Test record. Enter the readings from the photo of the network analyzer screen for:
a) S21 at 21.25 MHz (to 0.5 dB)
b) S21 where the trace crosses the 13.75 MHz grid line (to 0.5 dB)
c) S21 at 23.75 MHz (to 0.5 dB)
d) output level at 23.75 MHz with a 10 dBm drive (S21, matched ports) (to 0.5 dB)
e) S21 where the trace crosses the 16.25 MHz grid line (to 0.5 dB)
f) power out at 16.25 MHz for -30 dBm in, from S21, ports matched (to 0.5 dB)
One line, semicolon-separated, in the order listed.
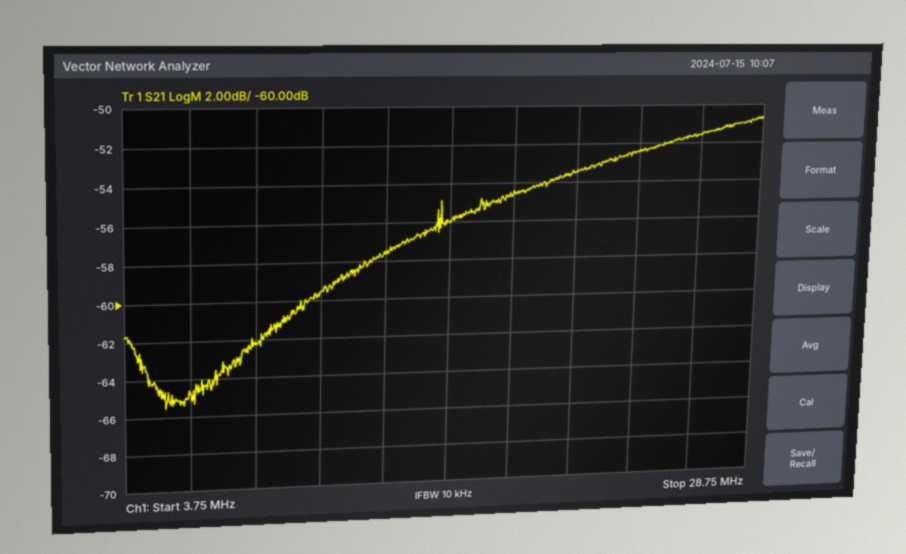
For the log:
-53.5 dB; -57.5 dB; -52.5 dB; -42.5 dBm; -56.0 dB; -86.0 dBm
